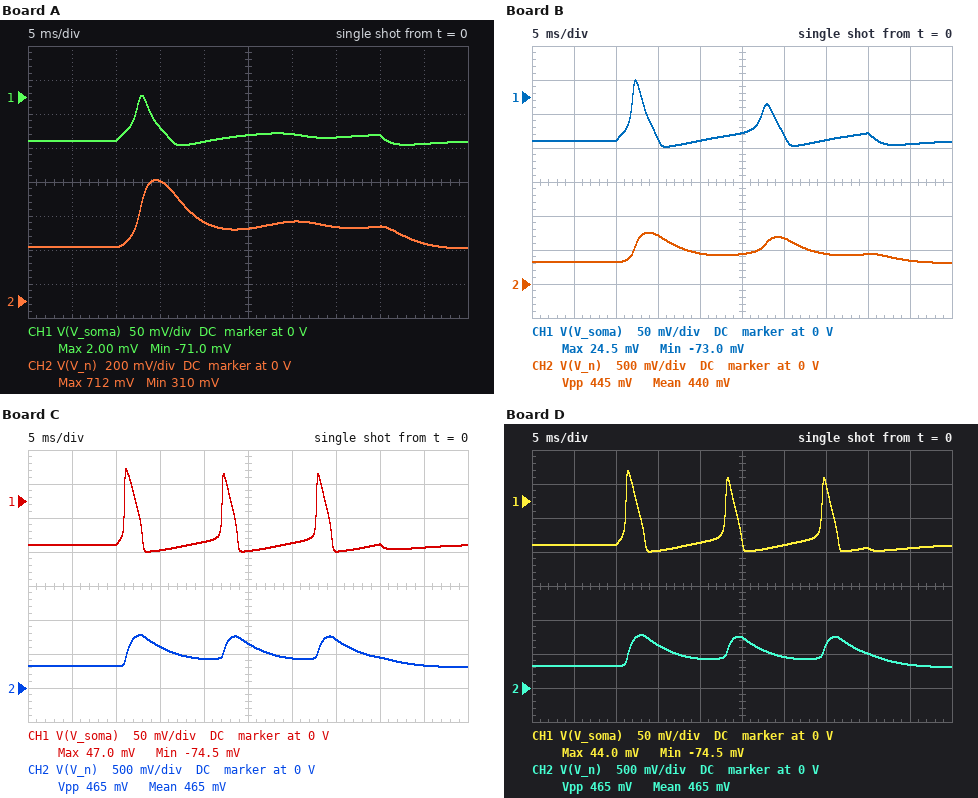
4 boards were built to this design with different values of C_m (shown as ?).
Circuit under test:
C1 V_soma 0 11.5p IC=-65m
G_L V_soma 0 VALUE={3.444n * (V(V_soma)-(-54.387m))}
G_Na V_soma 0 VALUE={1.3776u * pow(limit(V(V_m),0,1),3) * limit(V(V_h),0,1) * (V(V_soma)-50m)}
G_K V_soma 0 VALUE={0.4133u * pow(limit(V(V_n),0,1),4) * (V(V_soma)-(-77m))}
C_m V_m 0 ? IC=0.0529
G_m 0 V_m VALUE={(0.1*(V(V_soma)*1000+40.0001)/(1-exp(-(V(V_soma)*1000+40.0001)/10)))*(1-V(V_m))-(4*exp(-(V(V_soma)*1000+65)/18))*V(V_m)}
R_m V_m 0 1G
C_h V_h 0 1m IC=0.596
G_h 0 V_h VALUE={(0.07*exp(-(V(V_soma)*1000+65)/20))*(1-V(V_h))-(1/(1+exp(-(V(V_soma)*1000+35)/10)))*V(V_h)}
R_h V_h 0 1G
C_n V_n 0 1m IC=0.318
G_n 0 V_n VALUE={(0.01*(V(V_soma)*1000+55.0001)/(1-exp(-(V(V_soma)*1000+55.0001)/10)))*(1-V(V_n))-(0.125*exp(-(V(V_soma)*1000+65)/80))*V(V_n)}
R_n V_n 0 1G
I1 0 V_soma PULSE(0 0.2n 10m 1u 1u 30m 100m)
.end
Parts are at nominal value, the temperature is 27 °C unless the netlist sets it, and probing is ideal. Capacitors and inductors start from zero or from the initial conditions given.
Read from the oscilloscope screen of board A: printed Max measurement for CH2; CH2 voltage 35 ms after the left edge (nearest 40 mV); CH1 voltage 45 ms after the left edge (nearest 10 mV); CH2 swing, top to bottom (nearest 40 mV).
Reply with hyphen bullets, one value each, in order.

- 712 mV
- 440 mV
- -70 mV
- 400 mV
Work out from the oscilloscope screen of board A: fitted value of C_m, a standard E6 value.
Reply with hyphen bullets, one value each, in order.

- 3.3 mF
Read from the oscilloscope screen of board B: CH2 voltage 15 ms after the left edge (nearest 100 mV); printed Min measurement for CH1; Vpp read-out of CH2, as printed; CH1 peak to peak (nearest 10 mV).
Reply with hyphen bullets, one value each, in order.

- 700 mV
- -73.0 mV
- 445 mV
- 100 mV
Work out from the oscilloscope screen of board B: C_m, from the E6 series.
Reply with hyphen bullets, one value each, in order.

- 2.2 mF
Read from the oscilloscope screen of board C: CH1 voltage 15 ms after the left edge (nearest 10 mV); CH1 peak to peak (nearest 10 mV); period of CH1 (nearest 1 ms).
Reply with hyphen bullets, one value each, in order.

- -70 mV
- 120 mV
- 11 ms
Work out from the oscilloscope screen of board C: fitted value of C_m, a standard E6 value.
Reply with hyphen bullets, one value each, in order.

- 330 µF
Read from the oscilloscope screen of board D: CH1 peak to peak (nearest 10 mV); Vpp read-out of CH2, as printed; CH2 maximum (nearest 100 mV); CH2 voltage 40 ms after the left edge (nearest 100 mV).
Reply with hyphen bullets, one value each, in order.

- 120 mV
- 465 mV
- 800 mV
- 500 mV
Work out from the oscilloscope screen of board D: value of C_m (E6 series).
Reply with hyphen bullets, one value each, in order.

- 680 µF
